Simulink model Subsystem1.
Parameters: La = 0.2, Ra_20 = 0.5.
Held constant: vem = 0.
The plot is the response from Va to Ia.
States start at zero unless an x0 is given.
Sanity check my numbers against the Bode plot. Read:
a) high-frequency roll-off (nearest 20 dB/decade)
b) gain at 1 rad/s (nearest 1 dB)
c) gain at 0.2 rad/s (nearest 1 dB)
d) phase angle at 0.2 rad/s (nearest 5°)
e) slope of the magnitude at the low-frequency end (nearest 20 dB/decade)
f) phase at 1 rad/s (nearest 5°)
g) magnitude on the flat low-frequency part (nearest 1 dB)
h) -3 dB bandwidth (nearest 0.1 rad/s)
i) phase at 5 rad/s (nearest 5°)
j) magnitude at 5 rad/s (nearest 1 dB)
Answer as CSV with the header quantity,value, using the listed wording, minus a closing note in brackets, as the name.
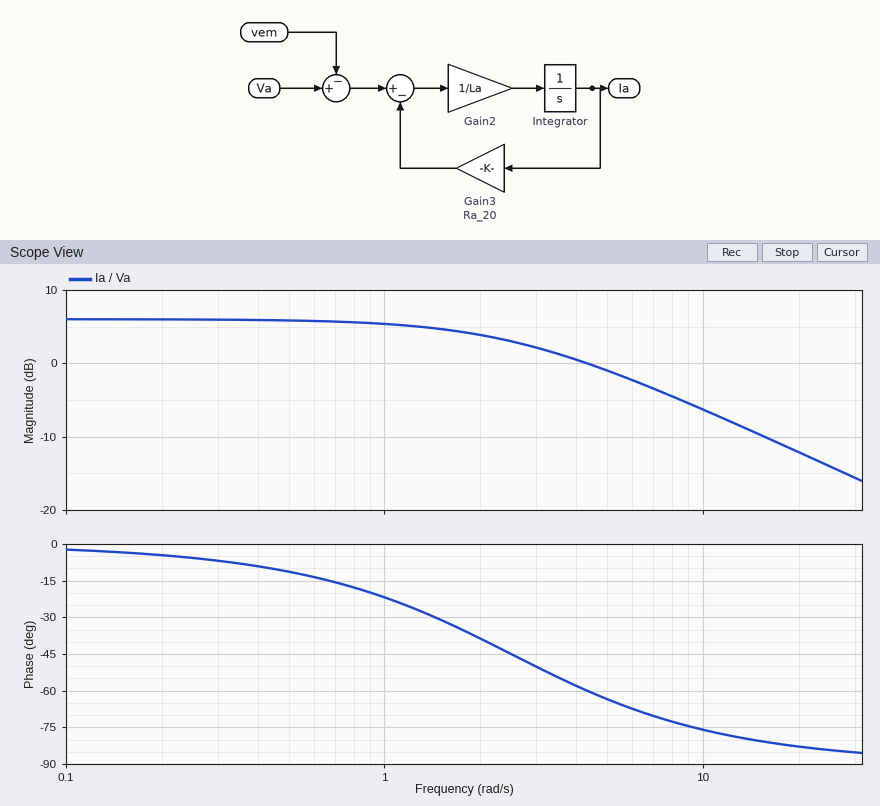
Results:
quantity,value
high-frequency roll-off,-20 dB/decade
gain at 1 rad/s,5 dB
gain at 0.2 rad/s,6 dB
phase angle at 0.2 rad/s,-5°
slope of the magnitude at the low-frequency end,0 dB/decade
phase at 1 rad/s,-20°
magnitude on the flat low-frequency part,6 dB
-3 dB bandwidth,2.5 rad/s
phase at 5 rad/s,-65°
magnitude at 5 rad/s,-1 dB
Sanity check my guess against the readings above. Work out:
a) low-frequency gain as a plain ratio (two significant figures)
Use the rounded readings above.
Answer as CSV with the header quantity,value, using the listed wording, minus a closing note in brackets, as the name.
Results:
quantity,value
low-frequency gain as a plain ratio,2.0
